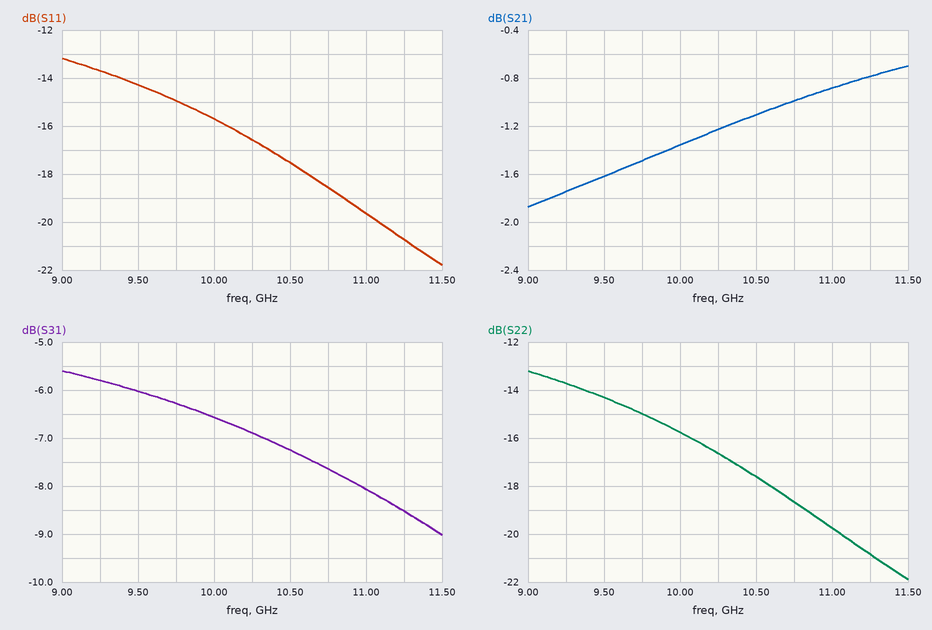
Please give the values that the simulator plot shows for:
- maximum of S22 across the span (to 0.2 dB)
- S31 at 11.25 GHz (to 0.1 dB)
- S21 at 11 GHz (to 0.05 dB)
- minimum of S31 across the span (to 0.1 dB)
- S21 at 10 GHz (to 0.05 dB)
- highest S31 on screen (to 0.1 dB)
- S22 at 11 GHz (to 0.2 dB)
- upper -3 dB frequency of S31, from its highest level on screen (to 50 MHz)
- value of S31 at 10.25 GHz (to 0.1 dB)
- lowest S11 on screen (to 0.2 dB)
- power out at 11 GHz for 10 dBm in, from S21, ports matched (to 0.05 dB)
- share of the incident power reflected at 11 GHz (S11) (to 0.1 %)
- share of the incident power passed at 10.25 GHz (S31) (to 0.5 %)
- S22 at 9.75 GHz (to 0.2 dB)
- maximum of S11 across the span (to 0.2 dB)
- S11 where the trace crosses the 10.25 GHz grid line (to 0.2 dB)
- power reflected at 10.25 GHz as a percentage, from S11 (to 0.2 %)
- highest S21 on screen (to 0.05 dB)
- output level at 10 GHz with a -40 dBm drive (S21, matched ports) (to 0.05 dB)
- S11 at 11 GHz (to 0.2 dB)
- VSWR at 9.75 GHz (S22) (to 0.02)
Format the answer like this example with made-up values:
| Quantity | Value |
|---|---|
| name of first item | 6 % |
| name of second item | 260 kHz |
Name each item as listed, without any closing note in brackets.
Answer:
| Quantity | Value |
|---|---|
| maximum of S22 across the span | -13.2 dB |
| S31 at 11.25 GHz | -8.5 dB |
| S21 at 11 GHz | -0.90 dB |
| minimum of S31 across the span | -9.0 dB |
| S21 at 10 GHz | -1.35 dB |
| highest S31 on screen | -5.6 dB |
| S22 at 11 GHz | -19.8 dB |
| upper -3 dB frequency of S31, from its highest level on screen | 11.30 GHz |
| value of S31 at 10.25 GHz | -6.9 dB |
| lowest S11 on screen | -21.8 dB |
| power out at 11 GHz for 10 dBm in, from S21, ports matched | 9.10 dBm |
| share of the incident power reflected at 11 GHz (S11) | 1.1 % |
| share of the incident power passed at 10.25 GHz (S31) | 20.5 % |
| S22 at 9.75 GHz | -15.0 dB |
| maximum of S11 across the span | -13.2 dB |
| S11 where the trace crosses the 10.25 GHz grid line | -16.6 dB |
| power reflected at 10.25 GHz as a percentage, from S11 | 2.2 % |
| highest S21 on screen | -0.70 dB |
| output level at 10 GHz with a -40 dBm drive (S21, matched ports) | -41.35 dBm |
| S11 at 11 GHz | -19.6 dB |
| VSWR at 9.75 GHz (S22) | 1.44 |
